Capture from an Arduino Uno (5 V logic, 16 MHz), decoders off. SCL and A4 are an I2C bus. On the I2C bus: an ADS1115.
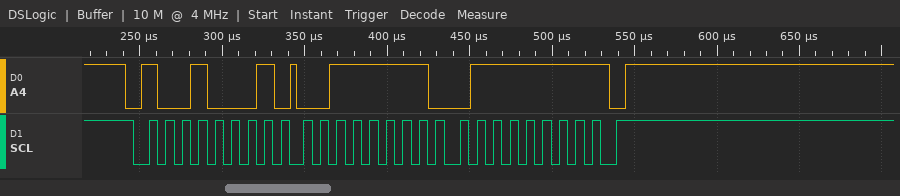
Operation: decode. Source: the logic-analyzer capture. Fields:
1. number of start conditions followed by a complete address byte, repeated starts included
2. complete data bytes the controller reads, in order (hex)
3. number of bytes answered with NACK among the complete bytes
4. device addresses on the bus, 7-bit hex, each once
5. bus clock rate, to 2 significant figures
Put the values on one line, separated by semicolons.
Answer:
1; 3F 7F; 1; 0x48; 100 kHz
